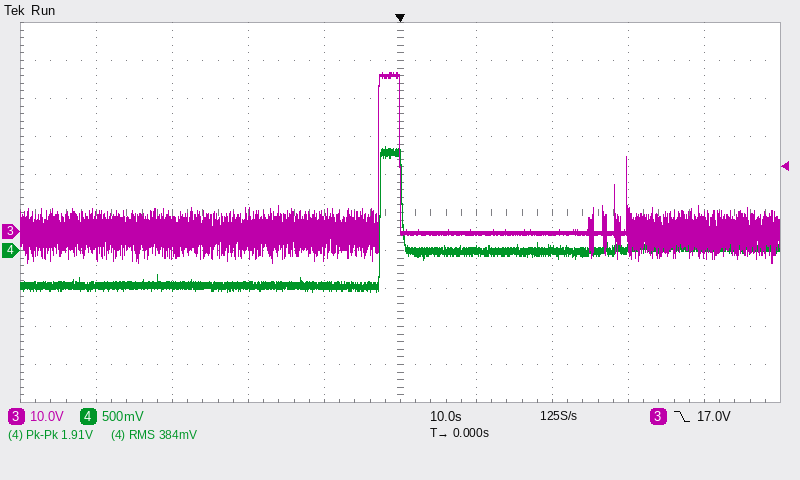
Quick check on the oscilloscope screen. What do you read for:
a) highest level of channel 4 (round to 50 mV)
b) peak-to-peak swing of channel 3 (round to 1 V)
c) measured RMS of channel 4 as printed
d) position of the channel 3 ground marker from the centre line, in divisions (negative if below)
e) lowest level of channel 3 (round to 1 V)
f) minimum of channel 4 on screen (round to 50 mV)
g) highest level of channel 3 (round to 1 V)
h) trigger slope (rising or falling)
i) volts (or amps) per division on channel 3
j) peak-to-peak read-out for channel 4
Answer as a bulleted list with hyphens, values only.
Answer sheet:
- 1.35 V
- 50 V
- 384 mV
- -0.5 div
- -8 V
- -550 mV
- 42 V
- falling
- 10 V
- 1.91 V
